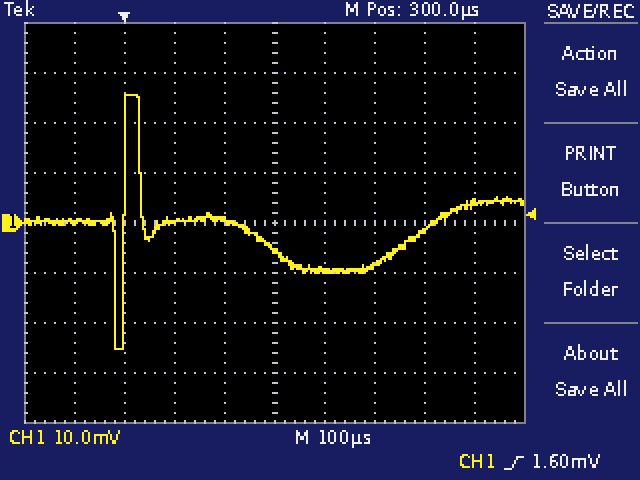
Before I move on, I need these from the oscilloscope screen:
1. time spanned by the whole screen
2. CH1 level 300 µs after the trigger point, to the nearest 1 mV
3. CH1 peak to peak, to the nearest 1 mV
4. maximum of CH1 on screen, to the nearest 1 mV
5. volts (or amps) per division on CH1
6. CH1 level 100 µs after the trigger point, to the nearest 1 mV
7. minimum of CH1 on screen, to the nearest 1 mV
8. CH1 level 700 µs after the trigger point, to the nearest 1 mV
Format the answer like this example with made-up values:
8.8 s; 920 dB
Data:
1 ms; -5 mV; 51 mV; 26 mV; 10 mV; 0 mV; -25 mV; 4 mV
